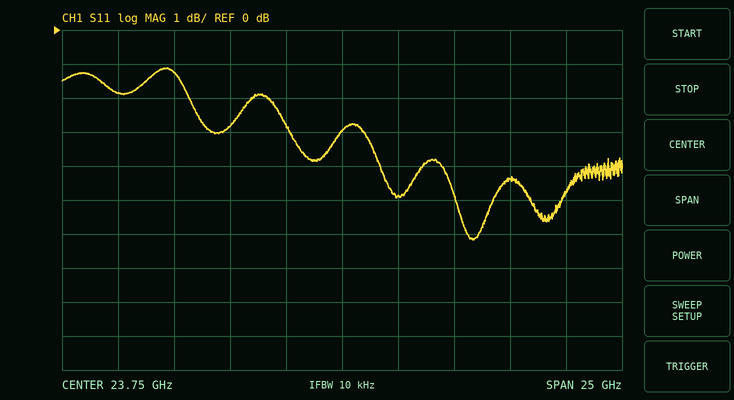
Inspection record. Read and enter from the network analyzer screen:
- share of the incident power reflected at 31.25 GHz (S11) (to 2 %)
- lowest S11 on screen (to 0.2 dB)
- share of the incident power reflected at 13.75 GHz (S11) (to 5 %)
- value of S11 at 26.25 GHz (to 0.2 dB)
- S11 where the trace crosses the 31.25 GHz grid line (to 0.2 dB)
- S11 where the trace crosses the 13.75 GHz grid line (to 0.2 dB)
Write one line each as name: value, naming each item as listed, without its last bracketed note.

share of the incident power reflected at 31.25 GHz (S11): 36 %
lowest S11 on screen: -6.2 dB
share of the incident power reflected at 13.75 GHz (S11): 65 %
value of S11 at 26.25 GHz: -4.8 dB
S11 where the trace crosses the 31.25 GHz grid line: -4.4 dB
S11 where the trace crosses the 13.75 GHz grid line: -1.8 dB
